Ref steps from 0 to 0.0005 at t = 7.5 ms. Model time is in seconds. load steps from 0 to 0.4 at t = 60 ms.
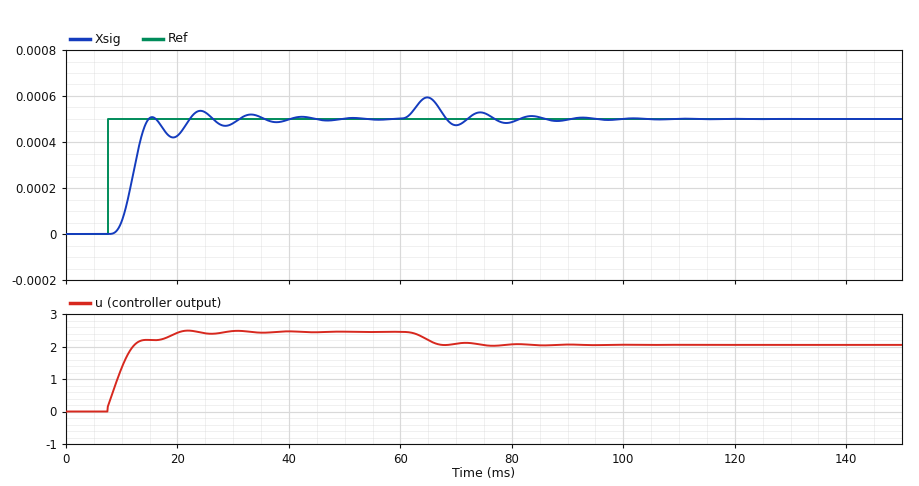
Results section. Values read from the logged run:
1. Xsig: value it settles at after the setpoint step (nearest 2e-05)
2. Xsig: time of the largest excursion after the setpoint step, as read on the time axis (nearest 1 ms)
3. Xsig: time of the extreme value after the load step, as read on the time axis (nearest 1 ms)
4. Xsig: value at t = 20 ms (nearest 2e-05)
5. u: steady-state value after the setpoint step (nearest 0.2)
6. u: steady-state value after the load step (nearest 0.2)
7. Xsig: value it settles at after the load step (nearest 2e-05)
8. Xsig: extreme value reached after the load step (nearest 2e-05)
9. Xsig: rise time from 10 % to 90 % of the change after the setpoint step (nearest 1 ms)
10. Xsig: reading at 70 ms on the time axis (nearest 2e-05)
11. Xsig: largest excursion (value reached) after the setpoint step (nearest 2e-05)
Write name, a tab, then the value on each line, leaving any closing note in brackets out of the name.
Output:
Xsig: value it settles at after the setpoint step	0.00050
Xsig: time of the largest excursion after the setpoint step, as read on the time axis	24 ms
Xsig: time of the extreme value after the load step, as read on the time axis	65 ms
Xsig: value at t = 20 ms	0.00042
u: steady-state value after the setpoint step	2.4
u: steady-state value after the load step	2.0
Xsig: value it settles at after the load step	0.00050
Xsig: extreme value reached after the load step	0.00060
Xsig: rise time from 10 % to 90 % of the change after the setpoint step	4 ms
Xsig: reading at 70 ms on the time axis	0.00048
Xsig: largest excursion (value reached) after the setpoint step	0.00054
